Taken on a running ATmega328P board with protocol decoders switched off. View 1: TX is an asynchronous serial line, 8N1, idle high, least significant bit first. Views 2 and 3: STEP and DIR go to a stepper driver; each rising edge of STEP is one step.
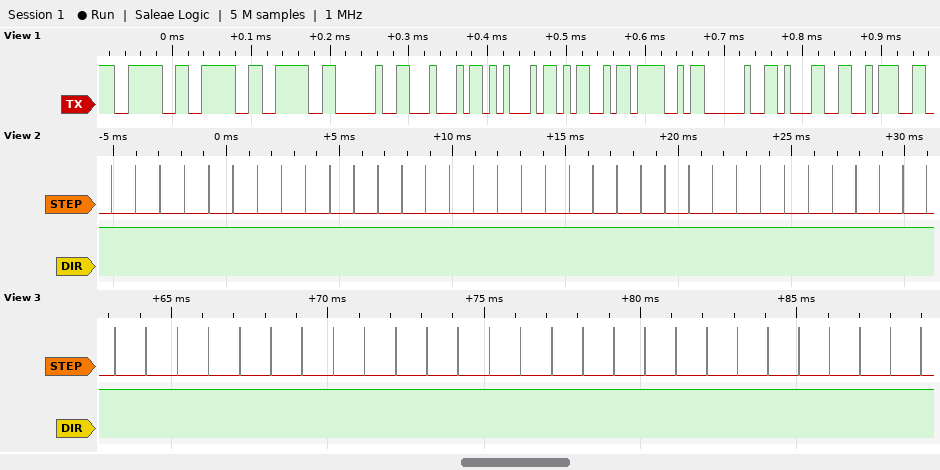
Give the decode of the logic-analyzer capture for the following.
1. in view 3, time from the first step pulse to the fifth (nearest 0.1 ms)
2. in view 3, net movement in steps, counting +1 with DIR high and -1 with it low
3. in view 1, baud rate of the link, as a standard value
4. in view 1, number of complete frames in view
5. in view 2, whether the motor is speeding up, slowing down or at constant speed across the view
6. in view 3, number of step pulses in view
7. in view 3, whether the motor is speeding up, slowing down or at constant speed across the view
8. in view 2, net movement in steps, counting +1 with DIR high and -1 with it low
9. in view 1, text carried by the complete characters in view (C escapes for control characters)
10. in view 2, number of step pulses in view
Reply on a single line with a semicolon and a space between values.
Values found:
4.0 ms; +27; 115200 baud; 11; constant speed; 27; constant speed; +35; ">>> DEMO 1:"; 35
